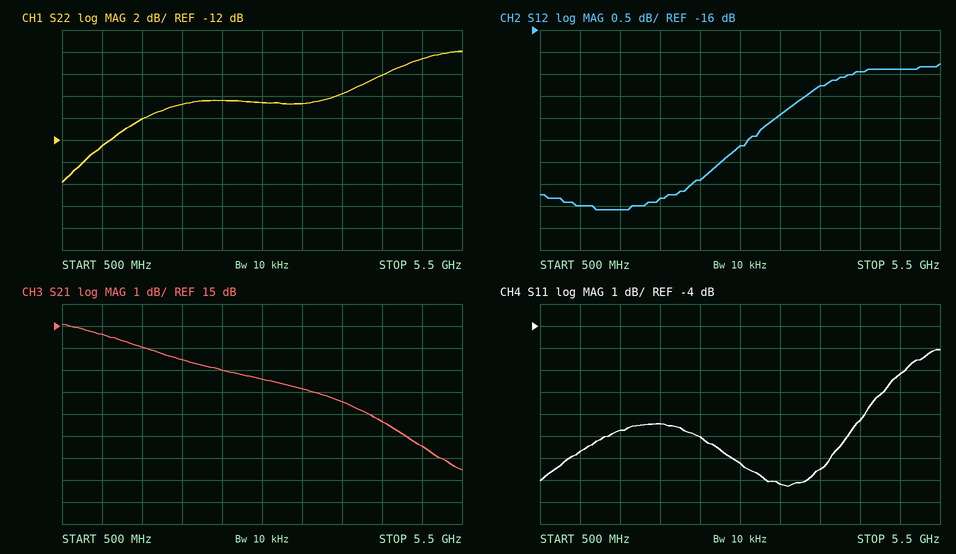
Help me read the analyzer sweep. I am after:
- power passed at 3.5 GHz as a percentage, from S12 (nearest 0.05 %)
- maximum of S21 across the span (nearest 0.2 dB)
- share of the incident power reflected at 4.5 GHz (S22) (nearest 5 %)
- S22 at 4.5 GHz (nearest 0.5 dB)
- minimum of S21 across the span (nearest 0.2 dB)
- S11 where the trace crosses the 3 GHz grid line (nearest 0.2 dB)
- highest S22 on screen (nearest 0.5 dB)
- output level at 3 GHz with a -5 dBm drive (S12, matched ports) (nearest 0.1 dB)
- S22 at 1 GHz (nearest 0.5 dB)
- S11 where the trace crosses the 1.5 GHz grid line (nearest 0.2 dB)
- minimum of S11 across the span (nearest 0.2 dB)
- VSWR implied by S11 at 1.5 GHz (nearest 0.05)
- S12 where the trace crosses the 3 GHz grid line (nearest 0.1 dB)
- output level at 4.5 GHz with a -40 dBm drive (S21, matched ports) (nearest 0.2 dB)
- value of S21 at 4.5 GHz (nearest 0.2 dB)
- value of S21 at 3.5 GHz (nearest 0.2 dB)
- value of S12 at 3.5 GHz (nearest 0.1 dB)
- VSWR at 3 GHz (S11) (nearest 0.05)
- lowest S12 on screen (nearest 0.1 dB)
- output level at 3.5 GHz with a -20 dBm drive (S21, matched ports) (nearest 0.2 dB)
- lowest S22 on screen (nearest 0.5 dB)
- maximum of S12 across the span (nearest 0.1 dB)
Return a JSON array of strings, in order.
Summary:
["1.60 %", "15.0 dB", "25 %", "-6.0 dB", "8.4 dB", "-10.2 dB", "-4.0 dB", "-23.6 dBm", "-12.5 dB", "-8.8 dB", "-11.2 dB", "2.15", "-18.6 dB", "-29.4 dBm", "10.6 dB", "12.2 dB", "-17.9 dB", "1.90", "-20.1 dB", "-7.8 dBm", "-16.0 dB", "-16.8 dB"]
